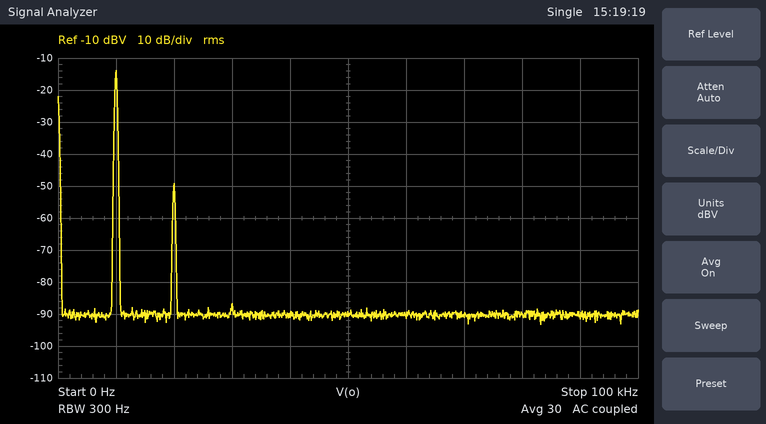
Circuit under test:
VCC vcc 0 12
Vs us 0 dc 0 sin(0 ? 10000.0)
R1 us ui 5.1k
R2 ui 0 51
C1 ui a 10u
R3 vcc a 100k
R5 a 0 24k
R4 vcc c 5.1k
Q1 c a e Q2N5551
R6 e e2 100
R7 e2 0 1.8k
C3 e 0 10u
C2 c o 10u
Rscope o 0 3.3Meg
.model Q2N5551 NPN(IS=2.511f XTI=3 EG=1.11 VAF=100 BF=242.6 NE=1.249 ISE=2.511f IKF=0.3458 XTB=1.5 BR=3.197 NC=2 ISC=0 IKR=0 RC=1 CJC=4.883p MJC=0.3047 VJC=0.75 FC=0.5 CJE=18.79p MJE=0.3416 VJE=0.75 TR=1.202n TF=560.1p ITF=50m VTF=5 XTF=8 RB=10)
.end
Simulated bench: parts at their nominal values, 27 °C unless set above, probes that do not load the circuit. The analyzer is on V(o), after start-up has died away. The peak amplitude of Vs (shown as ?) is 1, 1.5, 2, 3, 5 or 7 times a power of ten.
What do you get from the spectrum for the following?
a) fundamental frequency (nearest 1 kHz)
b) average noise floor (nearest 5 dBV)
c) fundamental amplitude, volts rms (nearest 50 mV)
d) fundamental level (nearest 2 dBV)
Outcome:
10 kHz
-90 dBV
200 mV
-14 dBV
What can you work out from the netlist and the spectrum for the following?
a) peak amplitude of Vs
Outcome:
200 mV
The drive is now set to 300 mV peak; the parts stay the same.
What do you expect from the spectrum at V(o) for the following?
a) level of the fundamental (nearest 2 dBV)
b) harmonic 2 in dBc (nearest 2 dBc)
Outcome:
-10 dBV
-32 dBc
